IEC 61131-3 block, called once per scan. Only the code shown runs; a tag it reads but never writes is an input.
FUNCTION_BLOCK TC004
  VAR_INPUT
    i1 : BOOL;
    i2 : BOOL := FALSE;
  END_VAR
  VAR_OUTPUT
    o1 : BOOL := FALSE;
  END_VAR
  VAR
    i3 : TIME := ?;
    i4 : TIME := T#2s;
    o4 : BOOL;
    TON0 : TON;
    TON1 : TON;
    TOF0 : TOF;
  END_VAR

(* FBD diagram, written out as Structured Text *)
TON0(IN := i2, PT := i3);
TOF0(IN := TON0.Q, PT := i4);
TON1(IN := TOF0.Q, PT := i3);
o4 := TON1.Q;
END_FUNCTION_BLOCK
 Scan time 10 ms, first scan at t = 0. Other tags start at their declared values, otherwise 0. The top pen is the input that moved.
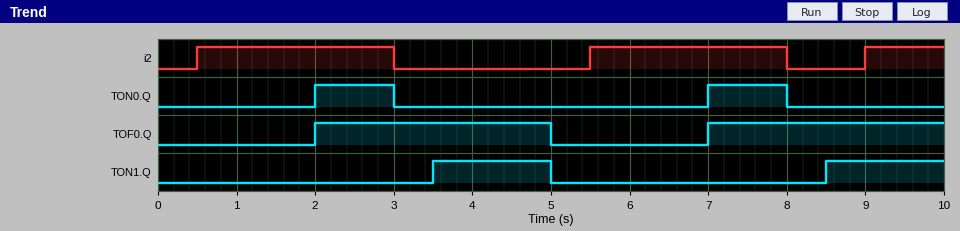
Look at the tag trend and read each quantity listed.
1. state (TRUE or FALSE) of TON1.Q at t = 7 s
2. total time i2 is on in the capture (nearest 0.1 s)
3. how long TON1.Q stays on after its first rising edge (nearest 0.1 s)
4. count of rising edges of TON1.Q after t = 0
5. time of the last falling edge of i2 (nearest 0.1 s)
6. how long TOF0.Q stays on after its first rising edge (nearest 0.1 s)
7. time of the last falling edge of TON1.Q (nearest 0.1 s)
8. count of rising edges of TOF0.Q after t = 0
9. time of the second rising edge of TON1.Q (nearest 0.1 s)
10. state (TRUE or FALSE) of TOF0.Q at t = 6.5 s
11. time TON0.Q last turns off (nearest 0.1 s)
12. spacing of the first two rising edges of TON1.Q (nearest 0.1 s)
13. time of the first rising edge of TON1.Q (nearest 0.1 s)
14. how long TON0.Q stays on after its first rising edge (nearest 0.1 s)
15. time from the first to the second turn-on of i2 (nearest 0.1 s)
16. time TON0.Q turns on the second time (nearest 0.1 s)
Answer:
FALSE
6.0 s
1.5 s
2
8.0 s
3.0 s
5.0 s
2
8.5 s
FALSE
8.0 s
5.0 s
3.5 s
1.0 s
5.0 s
7.0 s
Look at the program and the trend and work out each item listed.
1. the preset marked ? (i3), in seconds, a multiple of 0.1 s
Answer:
1.5 s
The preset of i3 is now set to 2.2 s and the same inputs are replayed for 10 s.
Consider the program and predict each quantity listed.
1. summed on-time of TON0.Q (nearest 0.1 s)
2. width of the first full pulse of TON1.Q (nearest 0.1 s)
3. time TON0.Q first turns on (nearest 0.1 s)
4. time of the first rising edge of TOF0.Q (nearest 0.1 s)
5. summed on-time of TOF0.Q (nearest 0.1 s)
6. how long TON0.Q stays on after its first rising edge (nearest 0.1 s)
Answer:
0.6 s
0.1 s
2.7 s
2.7 s
4.6 s
0.3 s
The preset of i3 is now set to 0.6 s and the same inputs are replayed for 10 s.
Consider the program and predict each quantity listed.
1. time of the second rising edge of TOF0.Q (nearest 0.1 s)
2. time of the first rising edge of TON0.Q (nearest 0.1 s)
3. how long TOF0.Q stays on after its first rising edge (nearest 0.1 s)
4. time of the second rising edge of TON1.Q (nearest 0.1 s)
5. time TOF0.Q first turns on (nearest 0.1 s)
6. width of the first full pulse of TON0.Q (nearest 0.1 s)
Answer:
6.1 s
1.1 s
3.9 s
6.7 s
1.1 s
1.9 s
